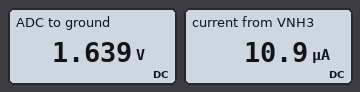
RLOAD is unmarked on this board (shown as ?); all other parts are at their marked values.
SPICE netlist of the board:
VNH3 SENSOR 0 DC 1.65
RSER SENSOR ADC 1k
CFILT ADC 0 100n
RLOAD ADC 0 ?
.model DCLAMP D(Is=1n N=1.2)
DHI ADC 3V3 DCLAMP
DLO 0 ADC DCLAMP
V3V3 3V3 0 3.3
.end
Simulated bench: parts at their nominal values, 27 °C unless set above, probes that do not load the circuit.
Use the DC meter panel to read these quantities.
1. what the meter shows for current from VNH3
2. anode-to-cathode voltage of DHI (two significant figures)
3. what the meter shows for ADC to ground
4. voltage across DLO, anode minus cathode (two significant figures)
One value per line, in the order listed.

10.9 µA
-1.7 V
1.639 V
-1.6 V
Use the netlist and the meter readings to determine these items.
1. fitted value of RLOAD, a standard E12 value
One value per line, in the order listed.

150 kΩ
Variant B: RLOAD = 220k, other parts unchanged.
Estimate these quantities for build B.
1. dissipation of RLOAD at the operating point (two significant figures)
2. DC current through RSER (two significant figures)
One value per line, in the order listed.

12 µW
7.5 µA
